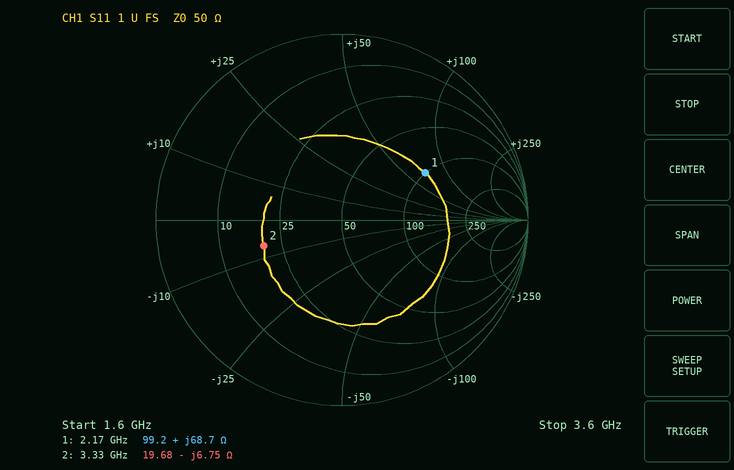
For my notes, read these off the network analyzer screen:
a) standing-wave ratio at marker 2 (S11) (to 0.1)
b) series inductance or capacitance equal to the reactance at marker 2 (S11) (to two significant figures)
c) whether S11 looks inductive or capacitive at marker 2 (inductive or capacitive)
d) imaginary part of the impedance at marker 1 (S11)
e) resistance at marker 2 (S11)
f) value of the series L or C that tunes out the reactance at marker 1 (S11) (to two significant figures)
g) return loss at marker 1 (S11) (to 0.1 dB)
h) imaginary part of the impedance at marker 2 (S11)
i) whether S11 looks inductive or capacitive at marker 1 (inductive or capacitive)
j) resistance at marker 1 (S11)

2.6
7.1 pF
capacitive
+68.7 Ω
19.68 Ω
1.1 pF
5.8 dB
-6.75 Ω
inductive
99.2 Ω
